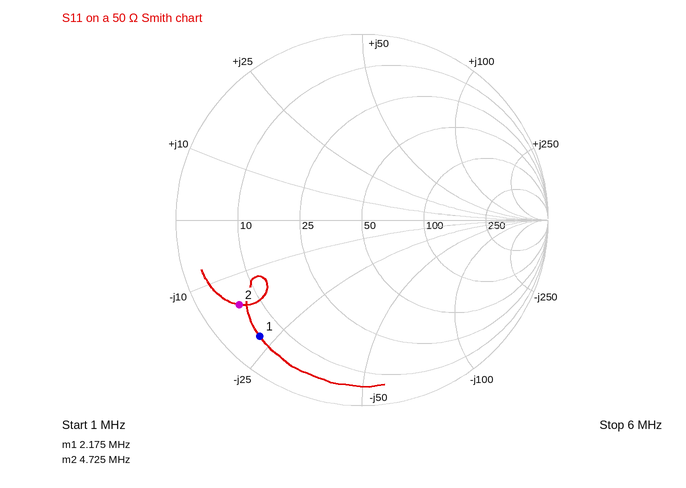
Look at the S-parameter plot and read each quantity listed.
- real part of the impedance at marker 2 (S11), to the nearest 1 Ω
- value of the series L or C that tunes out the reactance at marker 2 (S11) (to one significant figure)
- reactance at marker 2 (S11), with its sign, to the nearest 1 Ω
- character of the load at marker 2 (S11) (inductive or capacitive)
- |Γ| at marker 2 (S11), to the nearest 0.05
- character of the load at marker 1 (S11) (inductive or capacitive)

6 Ω
500 nH
-15 Ω
capacitive
0.80
capacitive
